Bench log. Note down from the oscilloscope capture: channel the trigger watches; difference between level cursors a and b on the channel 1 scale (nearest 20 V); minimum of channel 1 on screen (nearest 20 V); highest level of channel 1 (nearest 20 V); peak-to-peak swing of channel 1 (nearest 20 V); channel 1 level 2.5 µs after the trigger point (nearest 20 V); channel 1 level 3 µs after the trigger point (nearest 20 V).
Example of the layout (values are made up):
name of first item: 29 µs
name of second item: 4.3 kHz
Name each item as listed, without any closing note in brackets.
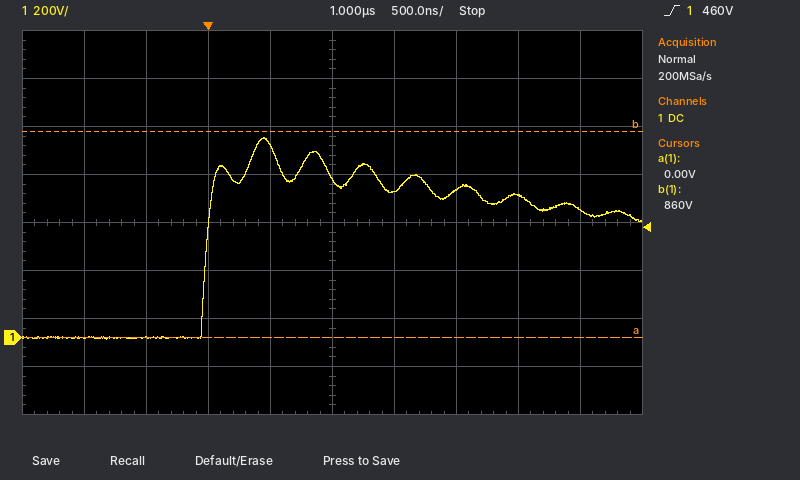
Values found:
channel the trigger watches: channel 1
difference between level cursors a and b on the channel 1 scale: 860 V
minimum of channel 1 on screen: 0 V
highest level of channel 1: 840 V
peak-to-peak swing of channel 1: 840 V
channel 1 level 2.5 µs after the trigger point: 600 V
channel 1 level 3 µs after the trigger point: 540 V
